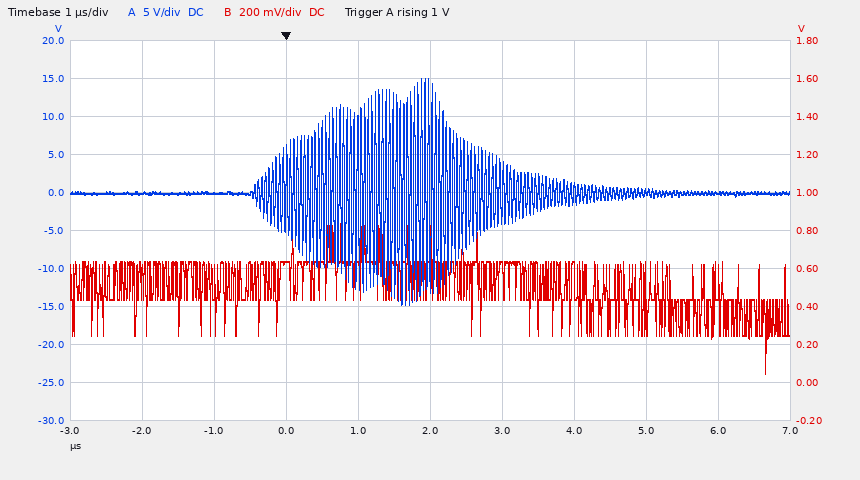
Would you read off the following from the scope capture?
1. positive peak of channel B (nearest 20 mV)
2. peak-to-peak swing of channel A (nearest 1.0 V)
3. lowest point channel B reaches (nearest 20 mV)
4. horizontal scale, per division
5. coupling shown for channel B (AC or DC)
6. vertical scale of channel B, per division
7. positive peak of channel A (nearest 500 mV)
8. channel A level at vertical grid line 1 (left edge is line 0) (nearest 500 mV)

840 mV
30.0 V
40 mV
1 µs
DC
200 mV
15.0 V
0.0 V
